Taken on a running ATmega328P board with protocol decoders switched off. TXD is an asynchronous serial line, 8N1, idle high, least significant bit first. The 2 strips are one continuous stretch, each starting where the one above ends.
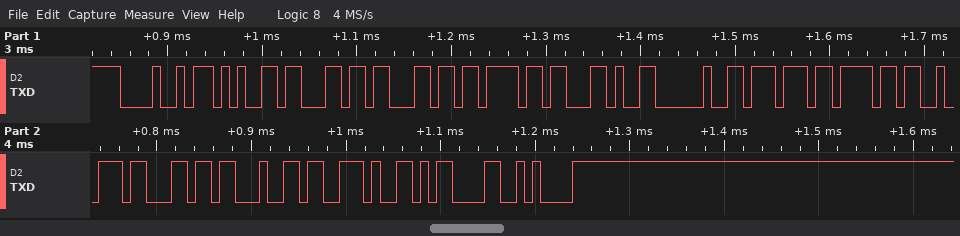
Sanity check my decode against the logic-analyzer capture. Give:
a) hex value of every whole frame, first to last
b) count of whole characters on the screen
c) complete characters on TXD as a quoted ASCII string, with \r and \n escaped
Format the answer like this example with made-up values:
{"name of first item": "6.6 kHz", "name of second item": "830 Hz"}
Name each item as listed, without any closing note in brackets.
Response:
{"hex value of every whole frame, first to last": "48 65 6C 6C 6F 2C 20 77 6F 72 6C 64 2E 0D 0A", "count of whole characters on the screen": "15", "complete characters on TXD as a quoted ASCII string, with \\r and \\n escaped": "\"Hello, world.\\r\\n\""}
